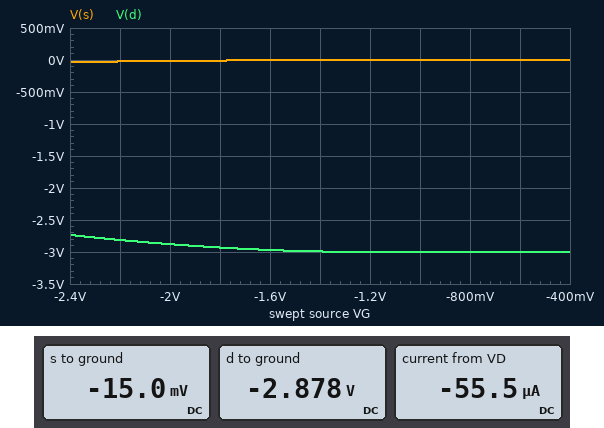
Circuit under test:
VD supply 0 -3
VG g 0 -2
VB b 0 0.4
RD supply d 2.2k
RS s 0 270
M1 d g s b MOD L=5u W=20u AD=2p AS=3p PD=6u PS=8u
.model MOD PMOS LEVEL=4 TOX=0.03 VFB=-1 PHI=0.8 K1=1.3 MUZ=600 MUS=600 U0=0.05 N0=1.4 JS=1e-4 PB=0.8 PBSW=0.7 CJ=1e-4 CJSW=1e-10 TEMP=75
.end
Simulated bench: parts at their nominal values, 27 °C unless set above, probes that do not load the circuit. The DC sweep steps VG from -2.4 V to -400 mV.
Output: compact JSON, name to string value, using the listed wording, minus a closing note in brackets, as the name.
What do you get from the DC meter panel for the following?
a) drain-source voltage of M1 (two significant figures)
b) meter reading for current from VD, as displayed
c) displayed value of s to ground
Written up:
{"drain-source voltage of M1": "-2.9 V", "meter reading for current from VD, as displayed": "-55.5 µA", "displayed value of s to ground": "-15.0 mV"}
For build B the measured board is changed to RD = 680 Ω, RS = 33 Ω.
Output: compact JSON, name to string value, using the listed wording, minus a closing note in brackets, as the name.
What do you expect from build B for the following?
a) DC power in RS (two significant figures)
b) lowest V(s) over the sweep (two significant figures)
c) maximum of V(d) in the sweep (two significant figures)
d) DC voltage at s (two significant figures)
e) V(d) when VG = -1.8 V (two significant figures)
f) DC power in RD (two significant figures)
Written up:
{"DC power in RS": "110 nW", "lowest V(s) over the sweep": "-4.3 mV", "maximum of V(d) in the sweep": "-2.9 V", "DC voltage at s": "-1.9 mV", "V(d) when VG = -1.8 V": "-3.0 V", "DC power in RD": "2.3 µW"}
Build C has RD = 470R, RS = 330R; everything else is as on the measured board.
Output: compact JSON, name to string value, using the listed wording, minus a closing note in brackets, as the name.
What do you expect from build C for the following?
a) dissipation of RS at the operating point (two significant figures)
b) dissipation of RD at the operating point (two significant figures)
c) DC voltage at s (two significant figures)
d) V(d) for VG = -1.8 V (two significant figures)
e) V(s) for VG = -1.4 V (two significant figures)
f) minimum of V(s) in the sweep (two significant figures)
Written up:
{"dissipation of RS at the operating point": "990 nW", "dissipation of RD at the operating point": "1.4 µW", "DC voltage at s": "-18 mV", "V(d) for VG = -1.8 V": "-3.0 V", "V(s) for VG = -1.4 V": "-1.3 mV", "minimum of V(s) in the sweep": "-39 mV"}
